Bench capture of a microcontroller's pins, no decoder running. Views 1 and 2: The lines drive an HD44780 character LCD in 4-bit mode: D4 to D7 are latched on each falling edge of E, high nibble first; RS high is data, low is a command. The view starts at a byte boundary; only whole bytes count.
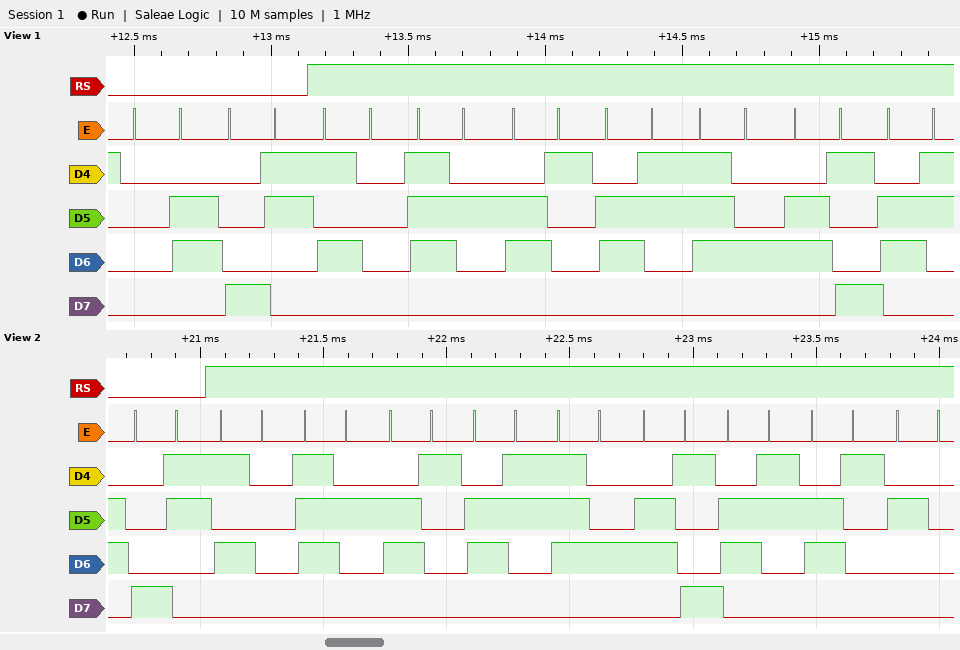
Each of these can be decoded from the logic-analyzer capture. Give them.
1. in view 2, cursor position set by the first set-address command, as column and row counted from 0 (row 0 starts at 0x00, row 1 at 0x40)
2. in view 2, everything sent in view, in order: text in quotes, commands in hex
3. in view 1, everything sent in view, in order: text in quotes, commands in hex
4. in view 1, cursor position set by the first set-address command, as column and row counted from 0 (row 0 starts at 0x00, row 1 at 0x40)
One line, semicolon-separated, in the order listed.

column 3, row 0; 0x83 "Practica "; 0x06 0x83 "Practic"; column 3, row 0
